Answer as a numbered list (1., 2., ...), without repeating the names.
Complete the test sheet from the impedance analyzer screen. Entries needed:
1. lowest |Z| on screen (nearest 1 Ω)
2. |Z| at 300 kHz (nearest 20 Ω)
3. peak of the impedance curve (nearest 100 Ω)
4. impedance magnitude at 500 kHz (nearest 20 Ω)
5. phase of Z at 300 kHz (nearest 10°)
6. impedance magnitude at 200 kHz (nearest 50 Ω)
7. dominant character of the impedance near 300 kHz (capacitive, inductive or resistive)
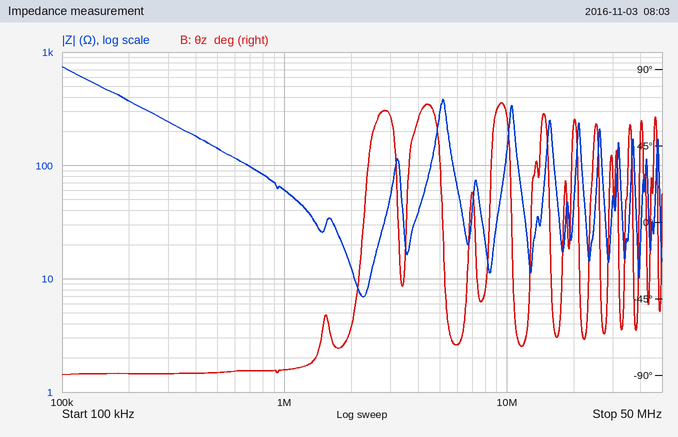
1. 7 Ω
2. 240 Ω
3. 700 Ω
4. 140 Ω
5. -90°
6. 350 Ω
7. capacitive
